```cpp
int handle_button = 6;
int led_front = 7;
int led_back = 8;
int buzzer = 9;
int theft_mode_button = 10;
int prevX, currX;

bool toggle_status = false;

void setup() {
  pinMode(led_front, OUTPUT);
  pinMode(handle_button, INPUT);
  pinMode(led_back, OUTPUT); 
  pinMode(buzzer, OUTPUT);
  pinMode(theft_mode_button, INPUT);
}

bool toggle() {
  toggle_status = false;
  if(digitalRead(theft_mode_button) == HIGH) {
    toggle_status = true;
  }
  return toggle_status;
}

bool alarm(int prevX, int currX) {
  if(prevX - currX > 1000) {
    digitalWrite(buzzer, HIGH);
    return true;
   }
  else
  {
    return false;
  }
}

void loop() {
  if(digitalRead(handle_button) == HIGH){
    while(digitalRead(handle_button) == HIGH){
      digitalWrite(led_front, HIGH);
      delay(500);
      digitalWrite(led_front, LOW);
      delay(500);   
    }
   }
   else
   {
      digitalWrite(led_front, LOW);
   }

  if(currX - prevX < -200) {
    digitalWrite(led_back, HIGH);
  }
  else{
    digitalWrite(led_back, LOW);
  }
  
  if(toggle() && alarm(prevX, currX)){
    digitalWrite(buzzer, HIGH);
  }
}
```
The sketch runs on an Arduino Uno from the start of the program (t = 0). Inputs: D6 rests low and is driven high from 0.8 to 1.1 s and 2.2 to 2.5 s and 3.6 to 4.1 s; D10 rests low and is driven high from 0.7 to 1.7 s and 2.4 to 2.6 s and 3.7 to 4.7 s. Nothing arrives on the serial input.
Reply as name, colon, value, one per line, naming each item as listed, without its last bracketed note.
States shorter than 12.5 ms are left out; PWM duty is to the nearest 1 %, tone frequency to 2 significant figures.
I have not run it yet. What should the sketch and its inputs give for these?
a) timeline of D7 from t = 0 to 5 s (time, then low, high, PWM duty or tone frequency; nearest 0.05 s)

timeline of D7 from t = 0 to 5 s: 0 s low; 0.8 s high; 1.3 s low; 2.2 s high; 2.7 s low; 3.6 s high; 4.1 s low
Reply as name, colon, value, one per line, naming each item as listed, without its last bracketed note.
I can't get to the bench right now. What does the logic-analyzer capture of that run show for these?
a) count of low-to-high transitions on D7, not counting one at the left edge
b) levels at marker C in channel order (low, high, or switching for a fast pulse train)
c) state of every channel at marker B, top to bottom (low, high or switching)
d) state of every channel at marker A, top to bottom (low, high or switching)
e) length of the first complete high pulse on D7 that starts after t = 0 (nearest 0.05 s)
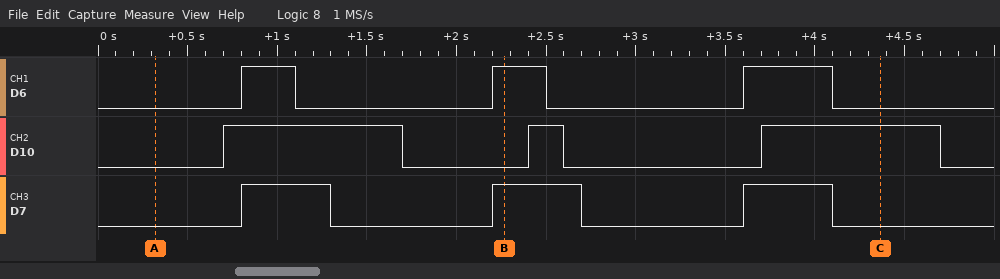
count of low-to-high transitions on D7, not counting one at the left edge: 3
levels at marker C in channel order: D6 low, D10 high, D7 low
state of every channel at marker B, top to bottom: D6 high, D10 low, D7 high
state of every channel at marker A, top to bottom: D6 low, D10 low, D7 low
length of the first complete high pulse on D7 that starts after t = 0: 0.50 s
